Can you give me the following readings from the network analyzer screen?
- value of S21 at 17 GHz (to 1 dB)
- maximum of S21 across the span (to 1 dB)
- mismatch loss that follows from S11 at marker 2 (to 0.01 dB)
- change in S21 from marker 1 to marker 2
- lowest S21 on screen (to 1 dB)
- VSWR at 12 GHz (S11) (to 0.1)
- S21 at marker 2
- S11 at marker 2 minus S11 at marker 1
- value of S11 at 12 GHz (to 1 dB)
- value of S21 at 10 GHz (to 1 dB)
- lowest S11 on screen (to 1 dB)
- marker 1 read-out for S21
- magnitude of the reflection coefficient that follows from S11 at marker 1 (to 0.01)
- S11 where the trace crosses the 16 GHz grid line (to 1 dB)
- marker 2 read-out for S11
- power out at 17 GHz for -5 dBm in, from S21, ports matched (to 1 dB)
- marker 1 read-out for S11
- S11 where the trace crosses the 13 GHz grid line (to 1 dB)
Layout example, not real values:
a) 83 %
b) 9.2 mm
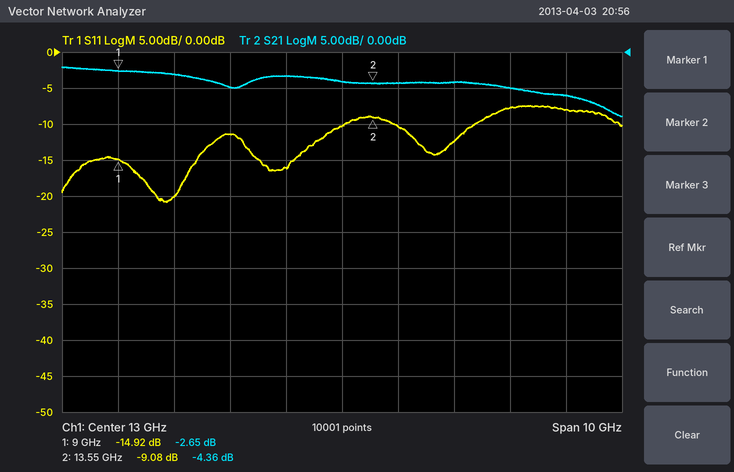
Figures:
a) -6 dB
b) -2 dB
c) 0.57 dB
d) -1.71 dB
e) -9 dB
f) 1.4
g) -4.36 dB
h) 5.84 dB
i) -16 dB
j) -3 dB
k) -21 dB
l) -2.65 dB
m) 0.18
n) -8 dB
o) -9.08 dB
p) -11 dBm
q) -14.92 dB
r) -10 dB
